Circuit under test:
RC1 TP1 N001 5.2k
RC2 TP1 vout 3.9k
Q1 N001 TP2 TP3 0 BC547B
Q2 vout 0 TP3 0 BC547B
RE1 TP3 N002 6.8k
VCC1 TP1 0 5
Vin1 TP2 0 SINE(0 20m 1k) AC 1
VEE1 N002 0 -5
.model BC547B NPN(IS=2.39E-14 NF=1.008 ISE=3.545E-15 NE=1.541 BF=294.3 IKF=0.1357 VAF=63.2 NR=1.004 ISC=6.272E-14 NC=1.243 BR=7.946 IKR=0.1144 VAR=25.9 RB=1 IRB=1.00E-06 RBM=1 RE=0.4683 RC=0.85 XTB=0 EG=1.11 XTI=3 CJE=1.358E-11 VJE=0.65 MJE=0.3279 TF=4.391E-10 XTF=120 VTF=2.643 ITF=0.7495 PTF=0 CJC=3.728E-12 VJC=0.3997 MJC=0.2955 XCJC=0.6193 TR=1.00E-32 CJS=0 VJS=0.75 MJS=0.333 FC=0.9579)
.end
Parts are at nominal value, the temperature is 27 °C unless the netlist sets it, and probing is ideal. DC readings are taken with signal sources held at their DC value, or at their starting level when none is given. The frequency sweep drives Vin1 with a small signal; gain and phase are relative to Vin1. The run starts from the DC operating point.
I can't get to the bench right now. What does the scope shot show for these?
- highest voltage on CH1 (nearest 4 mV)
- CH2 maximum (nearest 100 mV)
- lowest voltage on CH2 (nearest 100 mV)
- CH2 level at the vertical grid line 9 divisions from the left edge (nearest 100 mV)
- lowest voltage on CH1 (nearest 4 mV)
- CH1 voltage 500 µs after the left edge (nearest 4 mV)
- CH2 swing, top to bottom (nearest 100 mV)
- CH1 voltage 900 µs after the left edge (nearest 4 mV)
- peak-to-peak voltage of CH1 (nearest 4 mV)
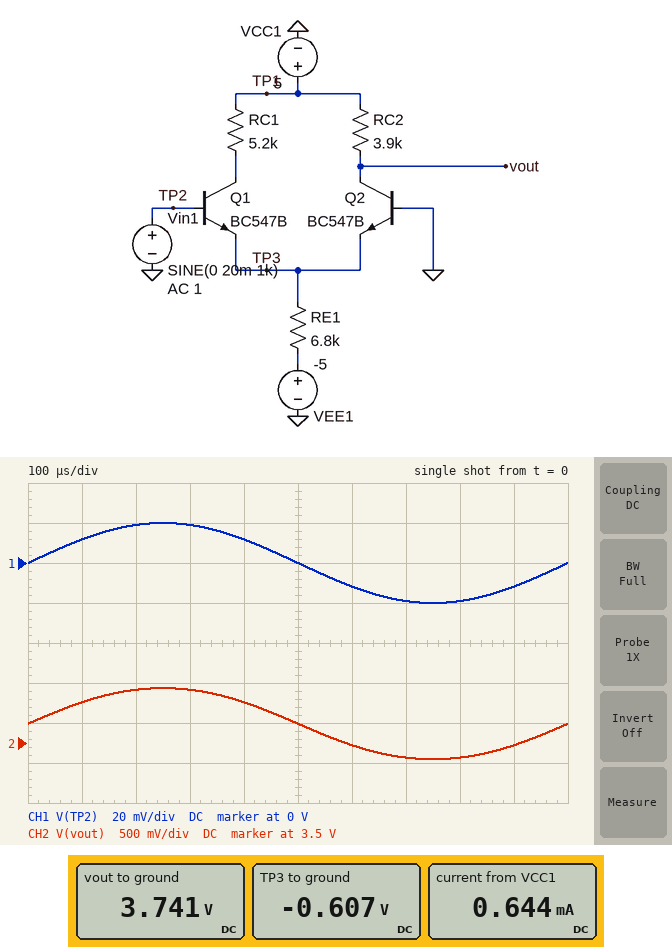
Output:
20 mV
4.2 V
3.3 V
3.5 V
-20 mV
0 V
900 mV
-12 mV
40 mV
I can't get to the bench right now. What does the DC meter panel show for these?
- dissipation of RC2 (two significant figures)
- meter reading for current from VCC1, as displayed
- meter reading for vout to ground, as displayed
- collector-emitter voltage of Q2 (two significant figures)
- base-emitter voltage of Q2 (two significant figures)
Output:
410 µW
0.644 mA
3.741 V
4.3 V
610 mV
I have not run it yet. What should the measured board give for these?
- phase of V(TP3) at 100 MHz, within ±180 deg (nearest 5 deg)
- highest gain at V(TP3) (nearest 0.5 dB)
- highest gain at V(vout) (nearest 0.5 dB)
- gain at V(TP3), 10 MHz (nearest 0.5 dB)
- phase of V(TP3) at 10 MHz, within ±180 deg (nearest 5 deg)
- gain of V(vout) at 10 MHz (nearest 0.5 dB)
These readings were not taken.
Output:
0 deg
-6.0 dB
27.5 dB
-6.0 dB
0 deg
26.5 dB
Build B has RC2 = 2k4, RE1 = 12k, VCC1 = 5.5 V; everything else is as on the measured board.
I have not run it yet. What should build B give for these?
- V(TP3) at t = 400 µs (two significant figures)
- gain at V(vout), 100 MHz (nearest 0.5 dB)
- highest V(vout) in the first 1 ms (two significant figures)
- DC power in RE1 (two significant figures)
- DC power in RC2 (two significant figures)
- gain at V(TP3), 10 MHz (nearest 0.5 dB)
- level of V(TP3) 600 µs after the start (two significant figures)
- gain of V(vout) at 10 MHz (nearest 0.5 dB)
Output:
-590 mV
9.5 dB
5.2 V
1.6 mW
81 µW
-6.0 dB
-600 mV
18.0 dB
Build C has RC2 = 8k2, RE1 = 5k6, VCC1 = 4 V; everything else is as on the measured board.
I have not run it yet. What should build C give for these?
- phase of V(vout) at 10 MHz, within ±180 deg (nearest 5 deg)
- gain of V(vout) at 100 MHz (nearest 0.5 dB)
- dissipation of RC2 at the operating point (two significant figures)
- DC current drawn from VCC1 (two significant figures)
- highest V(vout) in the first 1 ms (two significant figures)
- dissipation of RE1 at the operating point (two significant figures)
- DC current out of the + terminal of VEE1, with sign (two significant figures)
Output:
-55 deg
12.5 dB
1.2 mW
780 µA
1.9 V
3.4 mW
-780 µA
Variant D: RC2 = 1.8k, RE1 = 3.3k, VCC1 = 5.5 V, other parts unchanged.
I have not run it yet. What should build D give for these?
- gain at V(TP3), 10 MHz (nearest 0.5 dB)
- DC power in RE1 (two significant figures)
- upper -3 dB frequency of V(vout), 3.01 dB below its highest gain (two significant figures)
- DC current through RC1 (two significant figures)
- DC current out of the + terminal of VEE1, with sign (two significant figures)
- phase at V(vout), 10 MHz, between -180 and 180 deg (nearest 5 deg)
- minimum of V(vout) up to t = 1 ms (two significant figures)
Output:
-6.5 dB
5.8 mW
51 MHz
650 µA
-1.3 mA
-10 deg
3.9 V
